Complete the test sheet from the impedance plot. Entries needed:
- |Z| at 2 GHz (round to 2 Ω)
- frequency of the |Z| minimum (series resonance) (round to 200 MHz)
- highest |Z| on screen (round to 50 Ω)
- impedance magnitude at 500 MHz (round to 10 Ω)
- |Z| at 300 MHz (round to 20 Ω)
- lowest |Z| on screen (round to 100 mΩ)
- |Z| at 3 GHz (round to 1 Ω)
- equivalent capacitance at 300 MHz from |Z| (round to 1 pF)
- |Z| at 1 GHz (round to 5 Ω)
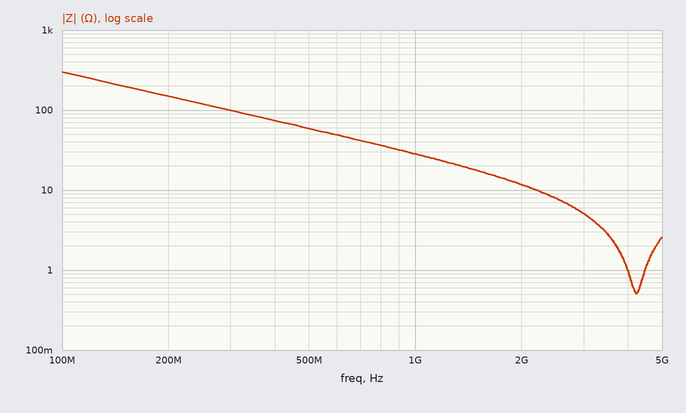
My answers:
12 Ω
4.2 GHz
300 Ω
60 Ω
100 Ω
500 mΩ
5 Ω
5 pF
30 Ω
